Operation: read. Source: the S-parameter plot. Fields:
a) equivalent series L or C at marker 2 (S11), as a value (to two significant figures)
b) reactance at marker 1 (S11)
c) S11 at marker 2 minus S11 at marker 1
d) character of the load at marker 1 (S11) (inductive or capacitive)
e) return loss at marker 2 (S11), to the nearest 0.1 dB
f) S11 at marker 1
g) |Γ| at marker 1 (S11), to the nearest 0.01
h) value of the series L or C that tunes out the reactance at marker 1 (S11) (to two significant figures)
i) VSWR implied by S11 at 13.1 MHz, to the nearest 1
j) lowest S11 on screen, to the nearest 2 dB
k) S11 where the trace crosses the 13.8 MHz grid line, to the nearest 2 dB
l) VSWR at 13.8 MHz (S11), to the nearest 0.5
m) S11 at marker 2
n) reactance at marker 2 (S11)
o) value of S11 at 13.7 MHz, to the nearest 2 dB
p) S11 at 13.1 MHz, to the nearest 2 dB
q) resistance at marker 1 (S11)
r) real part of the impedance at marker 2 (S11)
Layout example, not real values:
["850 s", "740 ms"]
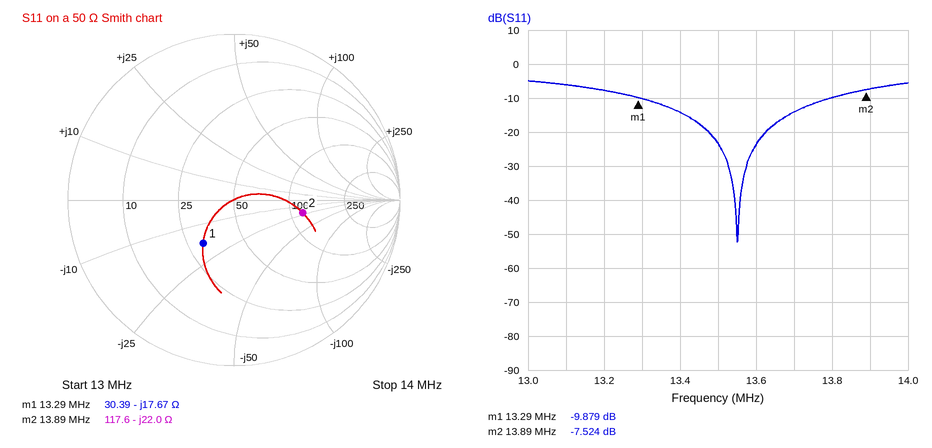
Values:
["520 pF", "-17.67 Ω", "2.355 dB", "capacitive", "7.5 dB", "-9.879 dB", "0.32", "210 nH", "3", "-52 dB", "-10 dB", "2.0", "-7.524 dB", "-22.0 Ω", "-14 dB", "-6 dB", "30.39 Ω", "117.6 Ω"]
